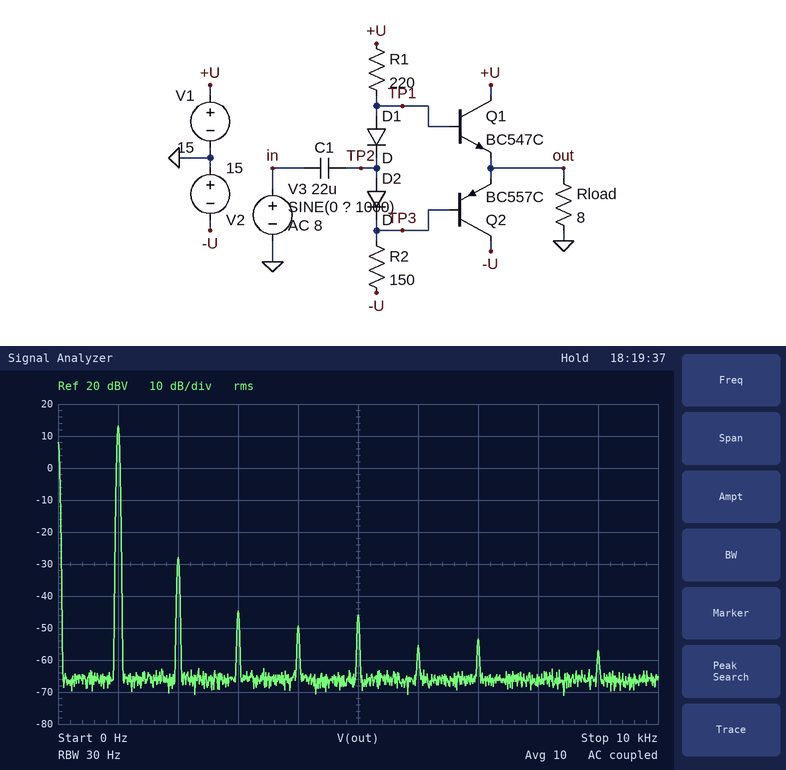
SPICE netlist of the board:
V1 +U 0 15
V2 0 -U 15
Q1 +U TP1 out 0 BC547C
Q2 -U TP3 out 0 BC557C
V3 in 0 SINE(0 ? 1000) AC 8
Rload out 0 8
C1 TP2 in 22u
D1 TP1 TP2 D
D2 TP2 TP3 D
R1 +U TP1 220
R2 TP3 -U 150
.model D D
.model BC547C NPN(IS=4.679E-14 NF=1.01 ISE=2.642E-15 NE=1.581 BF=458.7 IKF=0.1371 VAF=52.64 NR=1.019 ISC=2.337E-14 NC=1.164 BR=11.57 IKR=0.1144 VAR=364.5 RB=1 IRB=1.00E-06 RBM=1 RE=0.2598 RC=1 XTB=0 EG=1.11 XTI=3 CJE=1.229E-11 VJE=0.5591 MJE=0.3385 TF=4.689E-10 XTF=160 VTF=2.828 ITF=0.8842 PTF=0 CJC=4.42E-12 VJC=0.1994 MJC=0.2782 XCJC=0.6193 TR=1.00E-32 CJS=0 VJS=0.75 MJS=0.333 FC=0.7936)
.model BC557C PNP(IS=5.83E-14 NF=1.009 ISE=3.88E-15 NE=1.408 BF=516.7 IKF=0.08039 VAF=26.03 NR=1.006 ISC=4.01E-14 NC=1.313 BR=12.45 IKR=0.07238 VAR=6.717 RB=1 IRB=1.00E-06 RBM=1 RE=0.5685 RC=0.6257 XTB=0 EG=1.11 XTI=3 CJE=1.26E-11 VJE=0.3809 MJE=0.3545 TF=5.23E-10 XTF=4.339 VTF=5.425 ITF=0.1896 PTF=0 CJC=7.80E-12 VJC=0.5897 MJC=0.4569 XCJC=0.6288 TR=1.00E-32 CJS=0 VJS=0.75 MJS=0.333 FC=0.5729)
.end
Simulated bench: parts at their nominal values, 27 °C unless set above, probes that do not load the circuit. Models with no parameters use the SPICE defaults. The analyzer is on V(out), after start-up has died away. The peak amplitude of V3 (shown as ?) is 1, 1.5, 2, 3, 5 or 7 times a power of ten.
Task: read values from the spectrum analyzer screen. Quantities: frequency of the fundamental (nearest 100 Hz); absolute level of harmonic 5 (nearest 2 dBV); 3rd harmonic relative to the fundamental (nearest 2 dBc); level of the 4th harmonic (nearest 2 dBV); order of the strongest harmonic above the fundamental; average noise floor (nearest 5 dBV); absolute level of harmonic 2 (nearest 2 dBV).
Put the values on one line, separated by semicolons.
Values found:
1.0 kHz; -46 dBV; -58 dBc; -50 dBV; 2; -65 dBV; -28 dBV
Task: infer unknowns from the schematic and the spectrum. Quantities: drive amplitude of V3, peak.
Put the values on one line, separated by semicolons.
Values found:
7 V
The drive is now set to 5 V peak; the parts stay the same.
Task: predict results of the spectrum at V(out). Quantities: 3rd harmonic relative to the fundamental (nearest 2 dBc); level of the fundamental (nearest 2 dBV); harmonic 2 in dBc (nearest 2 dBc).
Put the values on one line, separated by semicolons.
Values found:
-52 dBc; 10 dBV; -42 dBc
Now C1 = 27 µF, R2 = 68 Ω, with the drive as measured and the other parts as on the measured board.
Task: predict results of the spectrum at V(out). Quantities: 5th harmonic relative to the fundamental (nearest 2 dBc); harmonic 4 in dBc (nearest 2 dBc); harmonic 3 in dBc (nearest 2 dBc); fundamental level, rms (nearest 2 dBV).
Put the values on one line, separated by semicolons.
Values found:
-52 dBc; -30 dBc; -24 dBc; 12 dBV
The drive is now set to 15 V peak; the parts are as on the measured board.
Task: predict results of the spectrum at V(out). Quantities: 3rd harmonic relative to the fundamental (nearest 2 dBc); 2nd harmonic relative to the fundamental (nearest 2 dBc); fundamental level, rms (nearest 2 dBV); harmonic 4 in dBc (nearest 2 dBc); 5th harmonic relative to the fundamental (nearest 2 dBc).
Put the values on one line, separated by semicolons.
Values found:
-18 dBc; -16 dBc; 18 dBV; -34 dBc; -46 dBc
